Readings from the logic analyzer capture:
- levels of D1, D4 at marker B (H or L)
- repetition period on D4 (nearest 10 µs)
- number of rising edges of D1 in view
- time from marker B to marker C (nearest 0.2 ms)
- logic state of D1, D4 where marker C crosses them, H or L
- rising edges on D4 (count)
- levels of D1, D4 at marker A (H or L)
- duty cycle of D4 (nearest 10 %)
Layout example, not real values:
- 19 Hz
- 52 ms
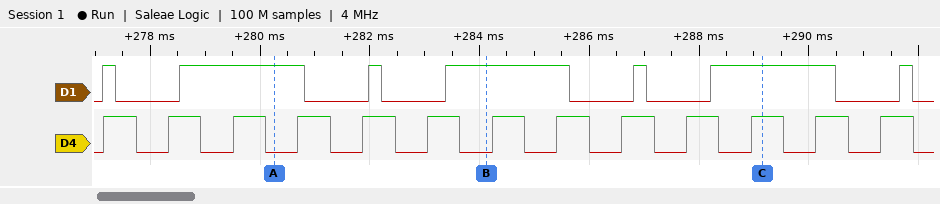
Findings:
- D1=H, D4=L
- 1180 µs
- 7
- 5 ms
- D1=H, D4=H
- 13
- D1=H, D4=L
- 50 %
